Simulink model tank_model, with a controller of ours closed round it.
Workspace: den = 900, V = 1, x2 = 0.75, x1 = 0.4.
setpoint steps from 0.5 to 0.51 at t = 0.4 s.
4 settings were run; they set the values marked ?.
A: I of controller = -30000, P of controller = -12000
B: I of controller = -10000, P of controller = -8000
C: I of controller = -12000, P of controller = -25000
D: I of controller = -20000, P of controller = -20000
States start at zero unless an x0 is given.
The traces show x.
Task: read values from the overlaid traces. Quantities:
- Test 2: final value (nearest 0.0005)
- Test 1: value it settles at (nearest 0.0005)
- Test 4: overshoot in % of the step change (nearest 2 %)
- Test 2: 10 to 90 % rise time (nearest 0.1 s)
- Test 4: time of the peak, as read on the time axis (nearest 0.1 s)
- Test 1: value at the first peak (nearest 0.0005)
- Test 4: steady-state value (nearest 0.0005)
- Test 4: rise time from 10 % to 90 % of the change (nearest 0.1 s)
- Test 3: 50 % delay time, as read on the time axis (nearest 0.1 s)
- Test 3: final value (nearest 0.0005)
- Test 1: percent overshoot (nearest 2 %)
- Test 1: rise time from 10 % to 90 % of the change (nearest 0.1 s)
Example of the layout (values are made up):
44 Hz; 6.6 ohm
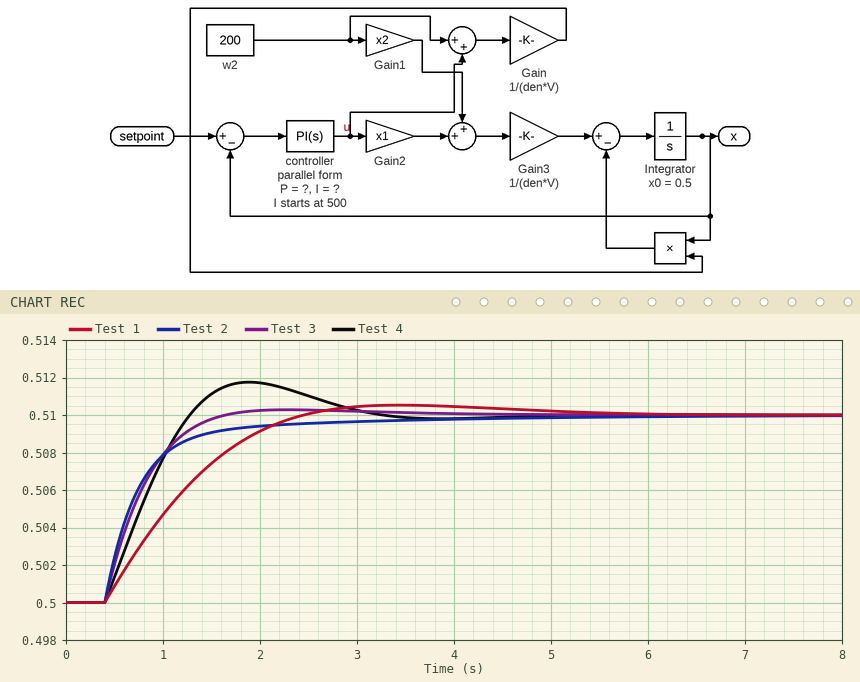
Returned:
0.5100; 0.5100; 18 %; 1.0 s; 1.9 s; 0.5105; 0.5100; 0.7 s; 0.7 s; 0.5100; 6 %; 1.4 s
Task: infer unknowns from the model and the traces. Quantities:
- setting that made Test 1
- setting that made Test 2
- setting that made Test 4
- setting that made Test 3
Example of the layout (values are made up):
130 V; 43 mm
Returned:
B; C; A; D
